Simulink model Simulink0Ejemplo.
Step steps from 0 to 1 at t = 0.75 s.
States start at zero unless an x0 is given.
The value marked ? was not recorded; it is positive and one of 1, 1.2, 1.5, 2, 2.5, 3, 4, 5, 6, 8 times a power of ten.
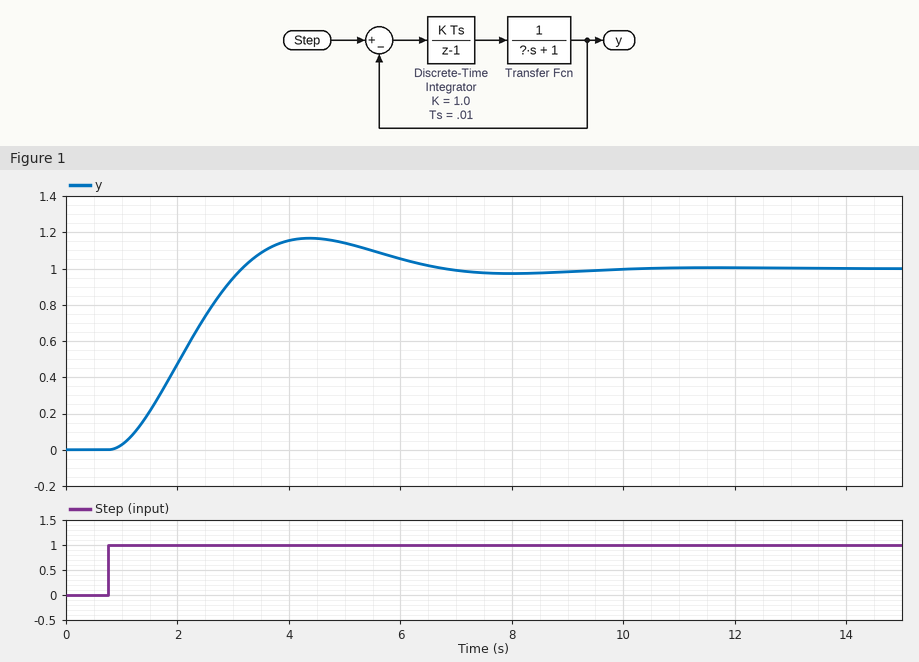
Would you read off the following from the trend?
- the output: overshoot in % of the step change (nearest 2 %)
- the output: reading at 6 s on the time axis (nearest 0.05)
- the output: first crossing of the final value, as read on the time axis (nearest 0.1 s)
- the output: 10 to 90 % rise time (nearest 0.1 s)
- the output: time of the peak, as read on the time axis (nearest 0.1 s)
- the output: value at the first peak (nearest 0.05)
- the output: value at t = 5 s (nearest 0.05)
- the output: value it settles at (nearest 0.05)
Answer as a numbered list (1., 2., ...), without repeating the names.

1. 16 %
2. 1.05
3. 3.2 s
4. 1.6 s
5. 4.4 s
6. 1.15
7. 1.15
8. 1.00
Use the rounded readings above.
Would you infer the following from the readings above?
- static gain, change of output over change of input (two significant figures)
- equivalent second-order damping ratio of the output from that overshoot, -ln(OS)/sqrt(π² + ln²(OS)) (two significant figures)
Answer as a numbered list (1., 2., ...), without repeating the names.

1. 1.0
2. 0.50
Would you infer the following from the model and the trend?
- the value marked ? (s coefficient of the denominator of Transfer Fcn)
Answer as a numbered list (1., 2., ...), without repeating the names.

1. 1
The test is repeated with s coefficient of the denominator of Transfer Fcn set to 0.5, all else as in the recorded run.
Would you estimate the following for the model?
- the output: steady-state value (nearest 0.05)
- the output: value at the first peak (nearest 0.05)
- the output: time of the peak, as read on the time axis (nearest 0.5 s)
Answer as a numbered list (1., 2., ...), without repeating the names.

1. 1.00
2. 1.05
3. 4.0 s
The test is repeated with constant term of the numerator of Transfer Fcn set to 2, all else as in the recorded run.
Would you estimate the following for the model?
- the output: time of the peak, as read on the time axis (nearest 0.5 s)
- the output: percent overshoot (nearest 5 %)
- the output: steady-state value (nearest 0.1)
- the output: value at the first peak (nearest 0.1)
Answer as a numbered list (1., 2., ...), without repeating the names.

1. 3.0 s
2. 30 %
3. 1.0
4. 1.3
